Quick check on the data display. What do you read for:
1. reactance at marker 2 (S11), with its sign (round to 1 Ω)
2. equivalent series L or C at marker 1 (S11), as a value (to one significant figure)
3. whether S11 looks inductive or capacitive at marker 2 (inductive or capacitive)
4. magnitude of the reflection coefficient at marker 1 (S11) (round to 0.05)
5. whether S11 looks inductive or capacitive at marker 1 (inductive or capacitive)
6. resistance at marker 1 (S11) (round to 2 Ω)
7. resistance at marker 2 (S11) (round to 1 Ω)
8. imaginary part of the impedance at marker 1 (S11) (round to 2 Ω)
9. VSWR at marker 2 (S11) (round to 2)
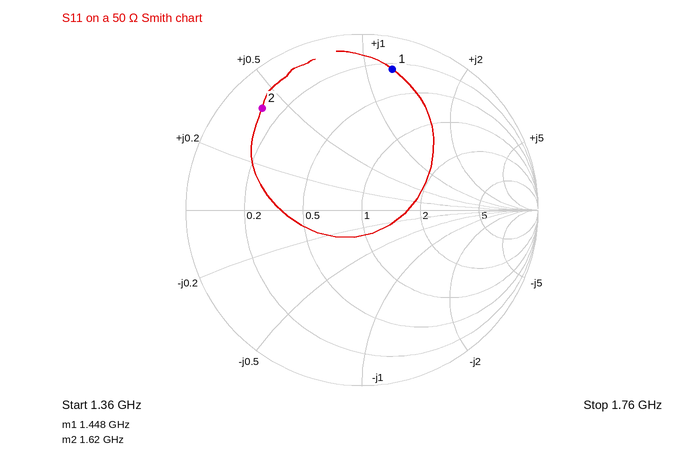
+21 Ω
7 nH
inductive
0.80
inductive
12 Ω
6 Ω
+60 Ω
10
